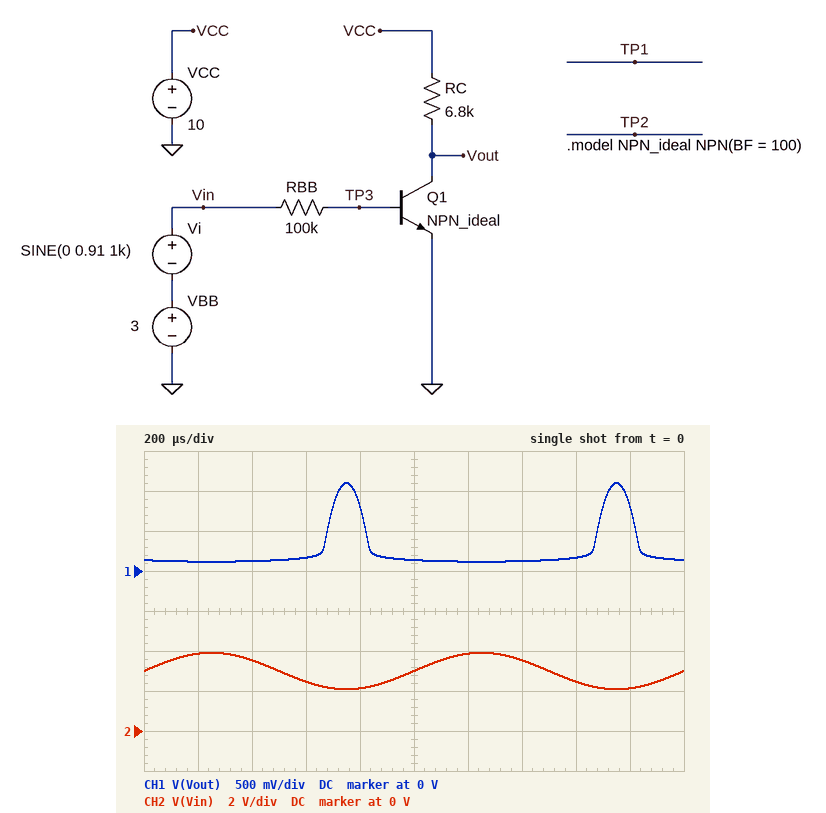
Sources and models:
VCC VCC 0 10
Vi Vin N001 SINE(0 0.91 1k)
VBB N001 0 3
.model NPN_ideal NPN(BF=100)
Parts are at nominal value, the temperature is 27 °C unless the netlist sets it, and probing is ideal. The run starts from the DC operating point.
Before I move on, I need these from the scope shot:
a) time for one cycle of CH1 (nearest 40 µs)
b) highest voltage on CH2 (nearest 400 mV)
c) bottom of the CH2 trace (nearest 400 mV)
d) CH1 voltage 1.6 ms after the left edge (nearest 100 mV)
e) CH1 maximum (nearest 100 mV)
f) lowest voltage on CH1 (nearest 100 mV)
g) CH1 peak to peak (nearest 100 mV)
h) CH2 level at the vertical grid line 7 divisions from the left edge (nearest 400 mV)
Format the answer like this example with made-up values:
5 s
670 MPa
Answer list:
1.00 ms
4.0 V
2.0 V
200 mV
1.1 V
100 mV
1.0 V
3.6 V
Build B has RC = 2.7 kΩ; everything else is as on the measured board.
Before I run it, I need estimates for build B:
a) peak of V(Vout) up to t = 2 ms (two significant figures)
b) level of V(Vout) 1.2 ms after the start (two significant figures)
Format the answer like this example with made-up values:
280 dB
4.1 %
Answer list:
6.5 V
1.7 V
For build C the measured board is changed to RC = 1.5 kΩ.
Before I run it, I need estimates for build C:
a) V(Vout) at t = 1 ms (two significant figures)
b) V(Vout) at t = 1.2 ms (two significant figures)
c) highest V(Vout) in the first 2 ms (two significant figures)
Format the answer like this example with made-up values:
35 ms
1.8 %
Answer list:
6.7 V
5.4 V
8.0 V
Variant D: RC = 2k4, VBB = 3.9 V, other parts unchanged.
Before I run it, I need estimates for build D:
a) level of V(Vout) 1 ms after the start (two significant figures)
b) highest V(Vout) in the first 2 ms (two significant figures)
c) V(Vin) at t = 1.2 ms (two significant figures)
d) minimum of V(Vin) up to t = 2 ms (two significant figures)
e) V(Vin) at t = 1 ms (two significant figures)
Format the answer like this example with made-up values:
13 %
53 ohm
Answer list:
2.6 V
4.7 V
4.8 V
3.0 V
3.9 V
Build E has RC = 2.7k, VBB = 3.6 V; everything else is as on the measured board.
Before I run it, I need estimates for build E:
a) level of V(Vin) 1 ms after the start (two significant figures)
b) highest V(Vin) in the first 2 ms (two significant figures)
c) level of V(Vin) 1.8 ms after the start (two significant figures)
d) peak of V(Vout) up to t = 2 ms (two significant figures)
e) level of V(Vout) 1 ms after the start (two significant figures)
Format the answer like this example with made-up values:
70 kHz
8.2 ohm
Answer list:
3.6 V
4.5 V
2.7 V
4.9 V
2.4 V
